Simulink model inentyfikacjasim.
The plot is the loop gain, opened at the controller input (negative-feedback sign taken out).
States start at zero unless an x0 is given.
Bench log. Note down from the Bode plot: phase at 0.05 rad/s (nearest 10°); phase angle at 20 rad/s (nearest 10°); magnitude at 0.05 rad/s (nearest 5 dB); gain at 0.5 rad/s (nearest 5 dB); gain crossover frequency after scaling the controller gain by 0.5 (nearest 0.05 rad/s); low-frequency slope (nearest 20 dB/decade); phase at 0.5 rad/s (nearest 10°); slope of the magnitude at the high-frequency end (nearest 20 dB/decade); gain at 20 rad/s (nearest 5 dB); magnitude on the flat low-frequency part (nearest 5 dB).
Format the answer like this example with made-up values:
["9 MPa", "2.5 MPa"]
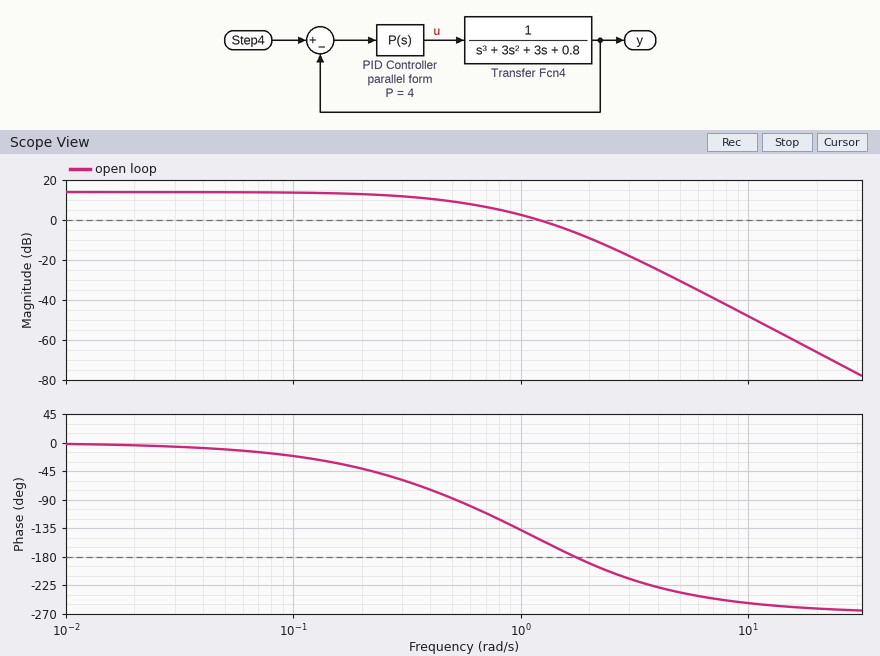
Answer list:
["-10°", "-260°", "15 dB", "10 dB", "0.75 rad/s", "0 dB/decade", "-90°", "-60 dB/decade", "-65 dB", "15 dB"]
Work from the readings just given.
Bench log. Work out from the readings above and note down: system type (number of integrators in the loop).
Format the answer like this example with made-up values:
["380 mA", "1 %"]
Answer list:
["0"]
